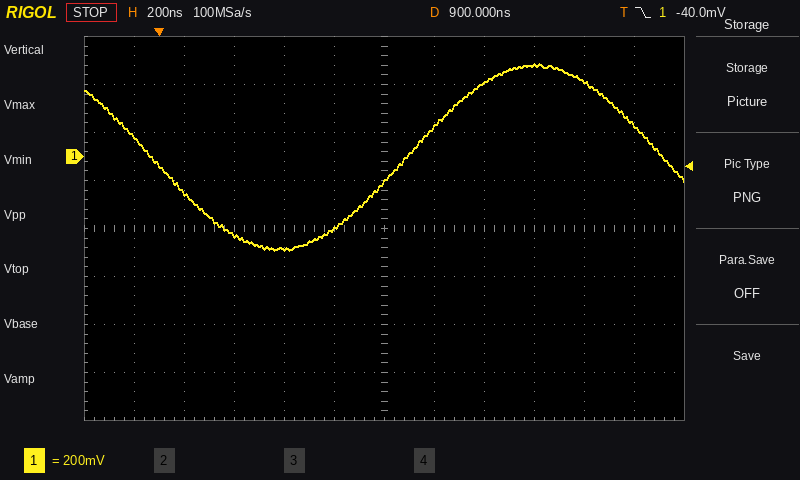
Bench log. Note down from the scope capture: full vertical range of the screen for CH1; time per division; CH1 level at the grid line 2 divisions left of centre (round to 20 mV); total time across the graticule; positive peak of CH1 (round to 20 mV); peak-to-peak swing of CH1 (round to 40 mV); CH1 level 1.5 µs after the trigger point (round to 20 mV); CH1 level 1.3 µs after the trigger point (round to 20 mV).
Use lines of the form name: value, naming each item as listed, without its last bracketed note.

full vertical range of the screen for CH1: 1.6 V
time per division: 200 ns
CH1 level at the grid line 2 divisions left of centre: -380 mV
total time across the graticule: 2.4 µs
positive peak of CH1: 380 mV
peak-to-peak swing of CH1: 760 mV
CH1 level 1.5 µs after the trigger point: 380 mV
CH1 level 1.3 µs after the trigger point: 300 mV
